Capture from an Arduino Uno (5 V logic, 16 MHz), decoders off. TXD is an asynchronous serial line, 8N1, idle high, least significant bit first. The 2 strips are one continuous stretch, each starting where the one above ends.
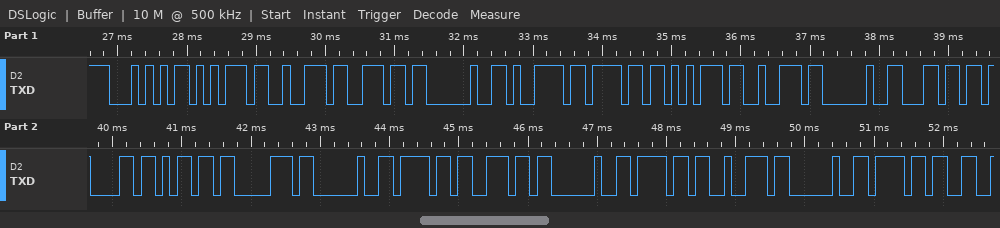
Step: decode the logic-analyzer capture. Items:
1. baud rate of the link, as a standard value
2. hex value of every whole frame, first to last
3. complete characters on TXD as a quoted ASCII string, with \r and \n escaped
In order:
9600 baud
0x54 0x75 0x72 0x6E 0x20 0x79 0x6F 0x75 0x72 0x20 0x6C 0x61 0x6D 0x70 0x20 0x6F 0x6E 0x20 0x6F 0x72 0x20 0x6F
"Turn your lamp on or o"
